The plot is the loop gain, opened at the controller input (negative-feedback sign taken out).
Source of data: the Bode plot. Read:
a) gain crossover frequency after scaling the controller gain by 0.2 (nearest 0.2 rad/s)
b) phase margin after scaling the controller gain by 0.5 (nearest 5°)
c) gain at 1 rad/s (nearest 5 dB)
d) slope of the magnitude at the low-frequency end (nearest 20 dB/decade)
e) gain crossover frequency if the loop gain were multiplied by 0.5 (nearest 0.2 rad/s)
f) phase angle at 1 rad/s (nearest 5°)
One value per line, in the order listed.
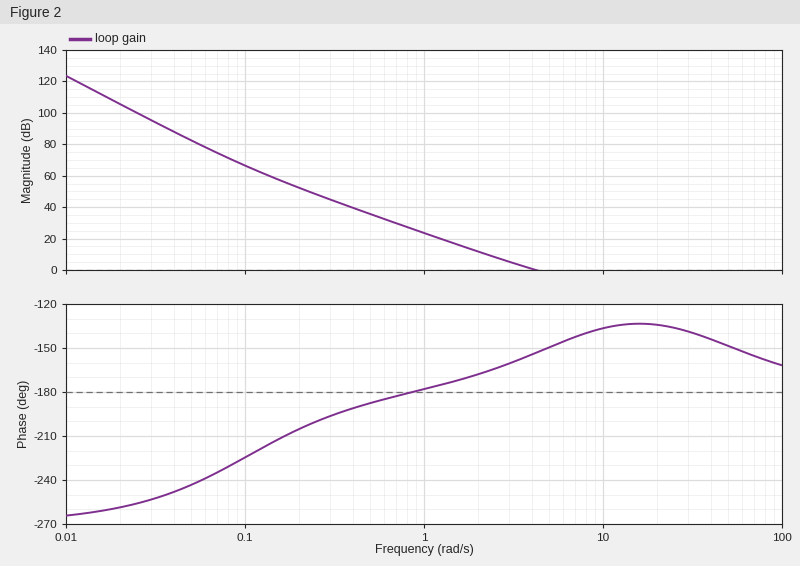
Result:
1.8 rad/s
20°
25 dB
-60 dB/decade
2.8 rad/s
-180°
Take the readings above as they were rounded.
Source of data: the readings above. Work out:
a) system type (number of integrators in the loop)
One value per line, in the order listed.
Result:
3
